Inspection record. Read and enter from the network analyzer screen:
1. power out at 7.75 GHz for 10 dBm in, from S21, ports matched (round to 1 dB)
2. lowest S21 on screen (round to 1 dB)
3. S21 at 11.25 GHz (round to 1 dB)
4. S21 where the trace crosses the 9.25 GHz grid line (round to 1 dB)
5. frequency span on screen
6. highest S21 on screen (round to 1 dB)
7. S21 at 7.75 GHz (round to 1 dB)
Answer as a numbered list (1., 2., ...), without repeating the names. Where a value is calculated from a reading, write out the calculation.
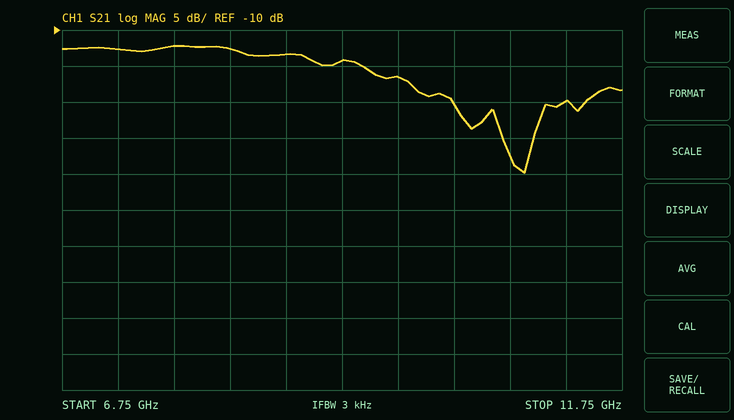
1. 10 dBm + (-12 dB) = -2 dBm
2. -30 dB
3. -20 dB
4. -14 dB
5. 5 GHz
6. -12 dB
7. -12 dB
